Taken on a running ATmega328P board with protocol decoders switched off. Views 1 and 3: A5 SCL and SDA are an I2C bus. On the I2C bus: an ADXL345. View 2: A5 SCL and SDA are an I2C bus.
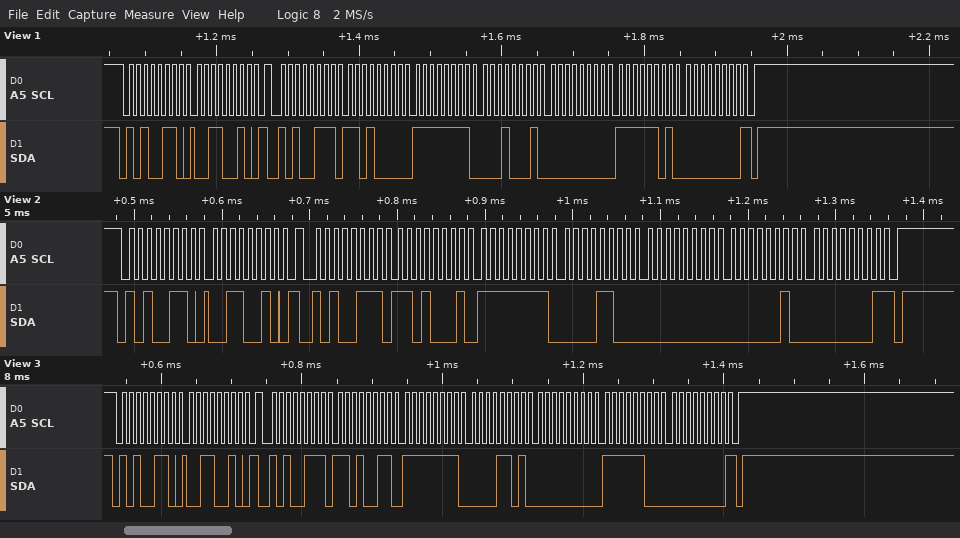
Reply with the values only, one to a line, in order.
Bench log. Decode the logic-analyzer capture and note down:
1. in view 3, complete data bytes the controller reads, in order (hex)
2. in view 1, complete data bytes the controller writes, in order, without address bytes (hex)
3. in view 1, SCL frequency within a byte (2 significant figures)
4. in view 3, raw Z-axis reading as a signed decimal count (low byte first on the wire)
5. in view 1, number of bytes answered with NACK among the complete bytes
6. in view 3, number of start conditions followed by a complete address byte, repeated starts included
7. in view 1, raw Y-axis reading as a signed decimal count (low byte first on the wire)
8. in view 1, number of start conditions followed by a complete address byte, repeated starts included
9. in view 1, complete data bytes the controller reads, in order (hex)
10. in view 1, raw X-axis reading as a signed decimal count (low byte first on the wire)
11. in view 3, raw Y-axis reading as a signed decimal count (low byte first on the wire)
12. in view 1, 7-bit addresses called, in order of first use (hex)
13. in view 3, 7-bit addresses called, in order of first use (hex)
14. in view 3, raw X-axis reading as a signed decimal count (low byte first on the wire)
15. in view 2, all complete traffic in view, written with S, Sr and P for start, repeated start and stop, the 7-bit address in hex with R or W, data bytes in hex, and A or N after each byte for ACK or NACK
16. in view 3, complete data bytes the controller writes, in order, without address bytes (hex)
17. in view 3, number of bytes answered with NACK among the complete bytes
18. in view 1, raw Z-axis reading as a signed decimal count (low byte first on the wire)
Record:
D3 FF 0D 00 FC 00
32
100 kHz
252
1
2
17
2
D0 FF 11 00 FD 00
-48
13
0x53
0x53
-45
S 53W A 32 A Sr 53R A D1 A FF A 0C A 00 A 02 A 01 N P
32
1
253
